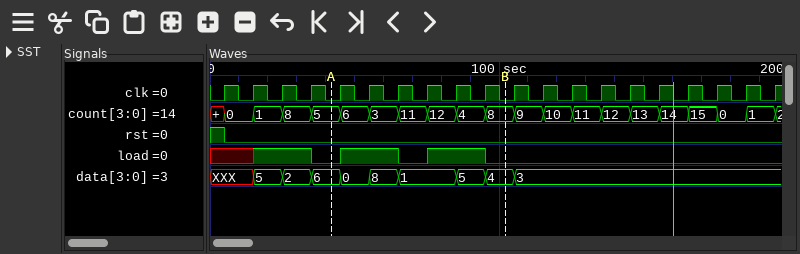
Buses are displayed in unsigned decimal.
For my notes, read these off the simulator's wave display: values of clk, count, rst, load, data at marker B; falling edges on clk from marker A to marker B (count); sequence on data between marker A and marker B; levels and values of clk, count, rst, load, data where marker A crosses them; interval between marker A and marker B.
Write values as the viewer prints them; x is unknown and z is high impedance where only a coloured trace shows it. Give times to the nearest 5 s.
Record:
clk=0, count=8, rst=0, load=0, data=4
6
6, 0, 8, 1, 5, 4
clk=0, count=5, rst=0, load=0, data=6
60 s
